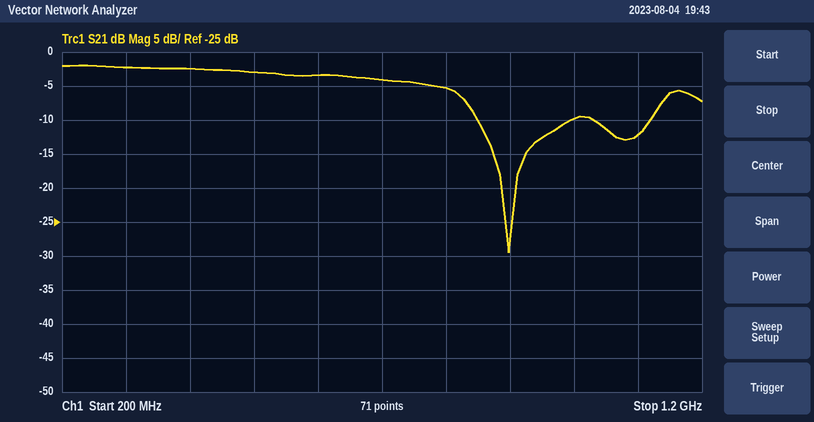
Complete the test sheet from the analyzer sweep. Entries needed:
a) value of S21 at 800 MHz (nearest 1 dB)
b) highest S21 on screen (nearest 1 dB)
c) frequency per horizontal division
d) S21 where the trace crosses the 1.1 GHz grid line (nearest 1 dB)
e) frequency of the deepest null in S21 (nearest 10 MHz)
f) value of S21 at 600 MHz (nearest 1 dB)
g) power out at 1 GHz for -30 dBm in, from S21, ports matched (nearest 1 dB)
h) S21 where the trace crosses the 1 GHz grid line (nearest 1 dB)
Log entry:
-5 dB
-2 dB
100 MHz
-12 dB
900 MHz
-3 dB
-40 dBm
-10 dB
